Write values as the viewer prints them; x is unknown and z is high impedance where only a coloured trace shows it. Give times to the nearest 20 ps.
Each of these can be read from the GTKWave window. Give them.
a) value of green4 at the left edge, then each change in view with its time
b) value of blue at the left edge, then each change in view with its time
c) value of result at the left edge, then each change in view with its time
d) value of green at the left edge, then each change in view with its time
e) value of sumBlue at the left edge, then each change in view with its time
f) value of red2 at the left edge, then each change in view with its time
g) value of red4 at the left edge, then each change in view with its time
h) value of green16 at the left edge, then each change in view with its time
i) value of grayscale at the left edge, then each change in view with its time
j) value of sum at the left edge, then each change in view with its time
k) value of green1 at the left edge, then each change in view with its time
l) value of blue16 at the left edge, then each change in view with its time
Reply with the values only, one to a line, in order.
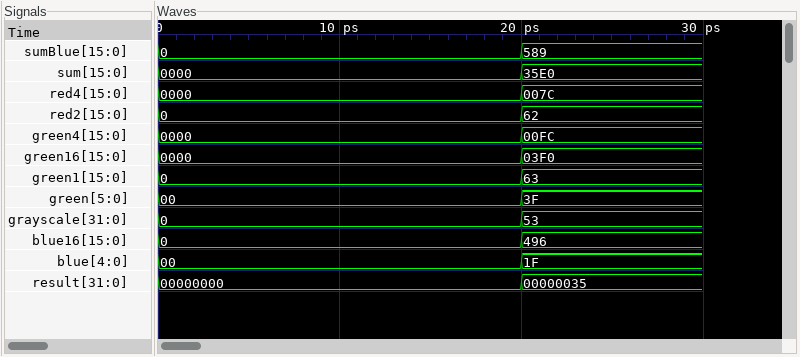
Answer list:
0000, 00FC at 20 ps
00, 1F at 20 ps
00000000, 00000035 at 20 ps
00, 3F at 20 ps
0, 589 at 20 ps
0, 62 at 20 ps
0000, 007C at 20 ps
0000, 03F0 at 20 ps
0, 53 at 20 ps
0000, 35E0 at 20 ps
0, 63 at 20 ps
0, 496 at 20 ps
